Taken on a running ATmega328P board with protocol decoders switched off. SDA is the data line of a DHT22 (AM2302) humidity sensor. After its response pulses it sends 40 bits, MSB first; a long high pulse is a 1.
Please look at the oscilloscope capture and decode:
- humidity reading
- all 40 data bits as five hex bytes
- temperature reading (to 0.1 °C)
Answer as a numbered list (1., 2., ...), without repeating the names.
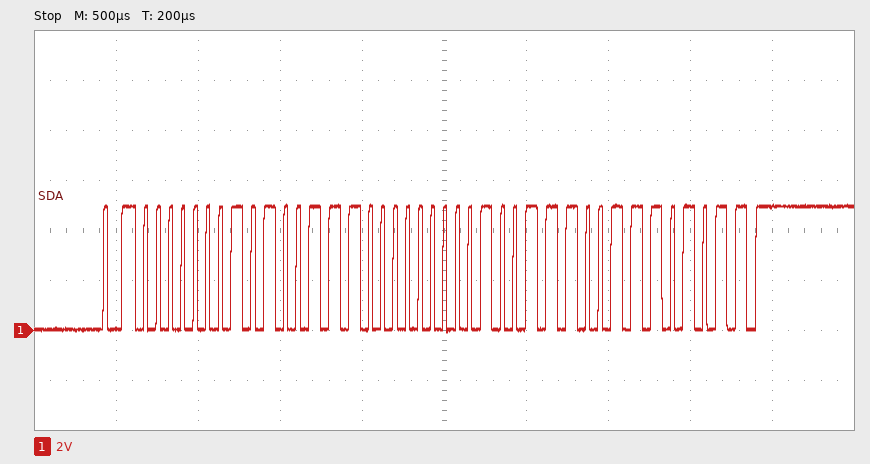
1. 33.4 %
2. 01 4E 00 9C EB
3. 15.6 °C
